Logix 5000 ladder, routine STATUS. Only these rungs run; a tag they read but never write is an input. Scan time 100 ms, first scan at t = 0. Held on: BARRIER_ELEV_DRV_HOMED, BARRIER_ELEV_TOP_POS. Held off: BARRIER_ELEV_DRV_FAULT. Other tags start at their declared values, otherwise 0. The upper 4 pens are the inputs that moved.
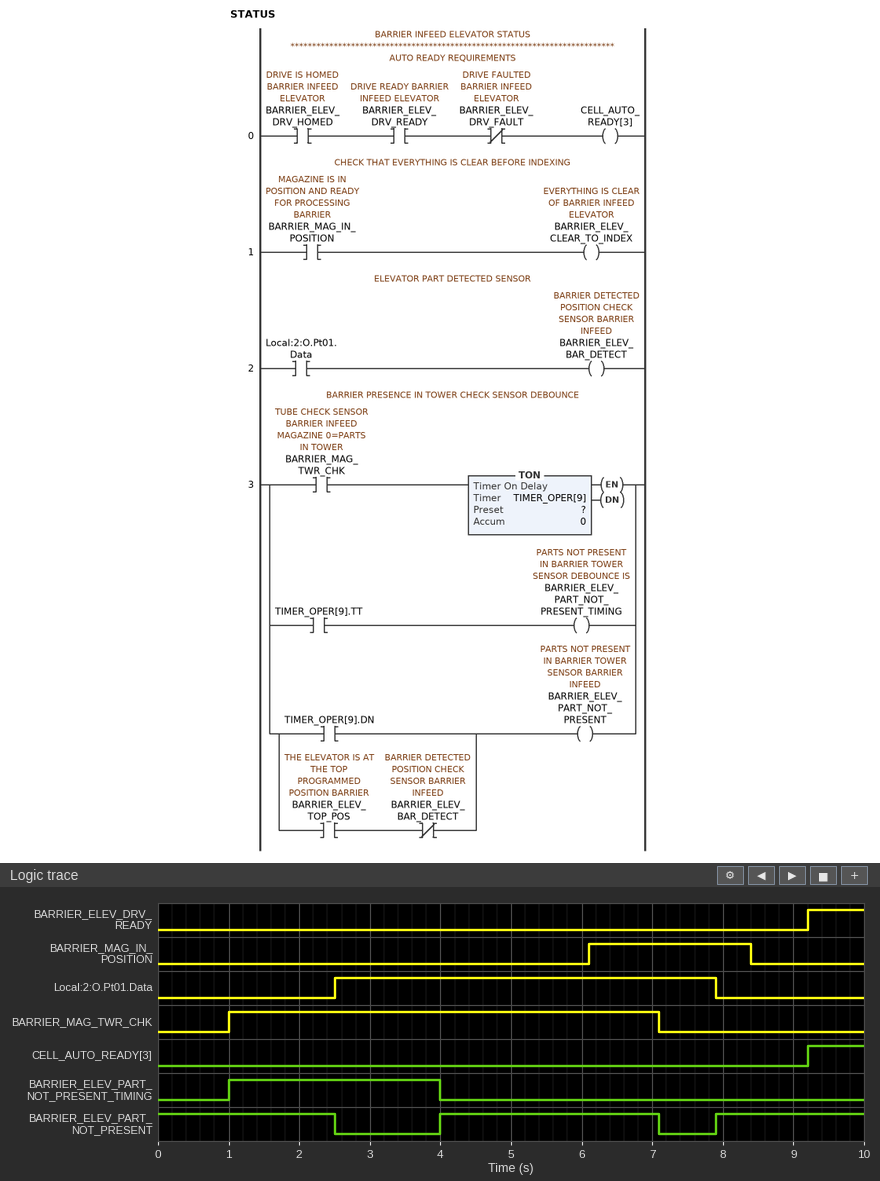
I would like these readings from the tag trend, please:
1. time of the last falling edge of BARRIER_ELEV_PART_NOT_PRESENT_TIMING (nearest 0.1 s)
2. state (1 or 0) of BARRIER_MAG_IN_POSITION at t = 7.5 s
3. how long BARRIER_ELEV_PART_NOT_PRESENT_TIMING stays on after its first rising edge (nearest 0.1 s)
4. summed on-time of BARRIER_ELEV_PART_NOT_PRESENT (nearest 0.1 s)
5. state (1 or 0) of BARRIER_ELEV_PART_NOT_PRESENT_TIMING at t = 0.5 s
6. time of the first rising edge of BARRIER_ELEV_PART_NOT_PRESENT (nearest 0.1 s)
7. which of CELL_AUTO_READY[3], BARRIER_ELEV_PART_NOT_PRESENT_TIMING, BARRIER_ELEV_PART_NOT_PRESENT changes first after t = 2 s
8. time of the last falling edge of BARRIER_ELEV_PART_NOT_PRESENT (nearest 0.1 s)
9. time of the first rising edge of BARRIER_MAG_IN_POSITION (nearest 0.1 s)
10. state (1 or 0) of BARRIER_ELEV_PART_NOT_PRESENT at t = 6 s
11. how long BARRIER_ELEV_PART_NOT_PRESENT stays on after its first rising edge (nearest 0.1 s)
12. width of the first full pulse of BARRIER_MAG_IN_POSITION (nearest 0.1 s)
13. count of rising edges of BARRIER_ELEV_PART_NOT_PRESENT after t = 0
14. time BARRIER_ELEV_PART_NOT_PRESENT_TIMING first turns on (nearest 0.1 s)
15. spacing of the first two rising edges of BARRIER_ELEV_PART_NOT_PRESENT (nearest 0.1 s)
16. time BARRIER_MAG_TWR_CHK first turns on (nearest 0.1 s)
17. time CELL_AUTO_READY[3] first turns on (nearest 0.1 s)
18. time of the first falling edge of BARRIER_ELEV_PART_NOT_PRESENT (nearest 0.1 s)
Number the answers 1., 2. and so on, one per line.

1. 4.0 s
2. 1
3. 3.0 s
4. 7.7 s
5. 0
6. 4.0 s
7. BARRIER_ELEV_PART_NOT_PRESENT
8. 7.1 s
9. 6.1 s
10. 1
11. 3.1 s
12. 2.3 s
13. 2
14. 1.0 s
15. 3.9 s
16. 1.0 s
17. 9.2 s
18. 2.5 s
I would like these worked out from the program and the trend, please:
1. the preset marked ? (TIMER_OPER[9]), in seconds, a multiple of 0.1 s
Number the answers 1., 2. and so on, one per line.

1. 3.0 s
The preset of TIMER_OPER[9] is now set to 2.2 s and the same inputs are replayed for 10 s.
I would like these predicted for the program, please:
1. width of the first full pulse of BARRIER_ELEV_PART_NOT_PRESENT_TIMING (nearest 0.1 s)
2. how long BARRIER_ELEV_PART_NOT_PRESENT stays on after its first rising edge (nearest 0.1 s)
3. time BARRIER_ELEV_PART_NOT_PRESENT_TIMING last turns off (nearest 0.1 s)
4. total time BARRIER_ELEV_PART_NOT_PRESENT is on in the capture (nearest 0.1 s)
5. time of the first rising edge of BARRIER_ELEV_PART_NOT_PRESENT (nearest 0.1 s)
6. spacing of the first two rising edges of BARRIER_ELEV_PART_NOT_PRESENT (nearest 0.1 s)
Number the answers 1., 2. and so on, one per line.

1. 2.2 s
2. 3.9 s
3. 3.2 s
4. 8.5 s
5. 3.2 s
6. 4.7 s
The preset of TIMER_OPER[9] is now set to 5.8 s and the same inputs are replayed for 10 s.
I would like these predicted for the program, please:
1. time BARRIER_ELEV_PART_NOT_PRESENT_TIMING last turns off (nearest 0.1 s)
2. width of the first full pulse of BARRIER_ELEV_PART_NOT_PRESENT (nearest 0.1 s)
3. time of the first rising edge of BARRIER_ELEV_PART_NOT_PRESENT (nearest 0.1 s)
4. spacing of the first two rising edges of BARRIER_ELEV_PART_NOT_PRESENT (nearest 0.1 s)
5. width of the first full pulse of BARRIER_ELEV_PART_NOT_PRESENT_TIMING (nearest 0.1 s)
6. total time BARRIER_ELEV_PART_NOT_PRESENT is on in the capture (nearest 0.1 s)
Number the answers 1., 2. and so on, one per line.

1. 6.8 s
2. 0.3 s
3. 6.8 s
4. 1.1 s
5. 5.8 s
6. 4.9 s
